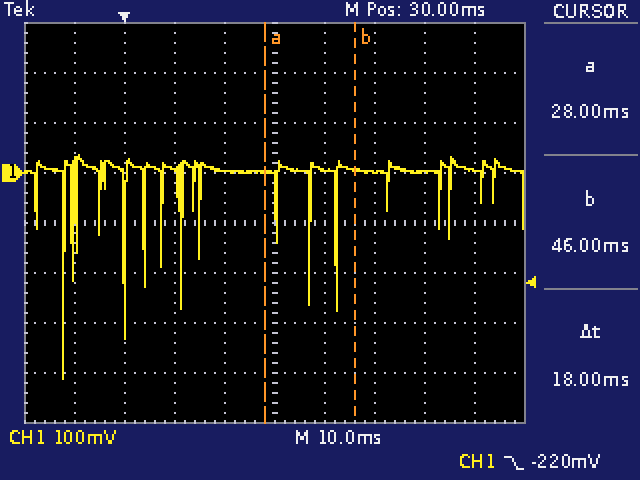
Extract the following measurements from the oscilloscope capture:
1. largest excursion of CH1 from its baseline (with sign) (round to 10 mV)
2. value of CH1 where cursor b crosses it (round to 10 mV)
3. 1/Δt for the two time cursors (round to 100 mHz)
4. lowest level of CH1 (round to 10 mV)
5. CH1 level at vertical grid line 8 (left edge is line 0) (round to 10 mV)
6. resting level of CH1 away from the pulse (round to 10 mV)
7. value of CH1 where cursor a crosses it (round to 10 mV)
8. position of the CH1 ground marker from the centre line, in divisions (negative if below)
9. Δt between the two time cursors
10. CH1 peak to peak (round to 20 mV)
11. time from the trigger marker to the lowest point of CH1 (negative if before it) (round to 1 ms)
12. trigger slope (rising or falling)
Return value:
-420 mV
10 mV
55.6 Hz
-410 mV
0 mV
10 mV
0 mV
+1.0 div
18 ms
440 mV
-12 ms
falling
